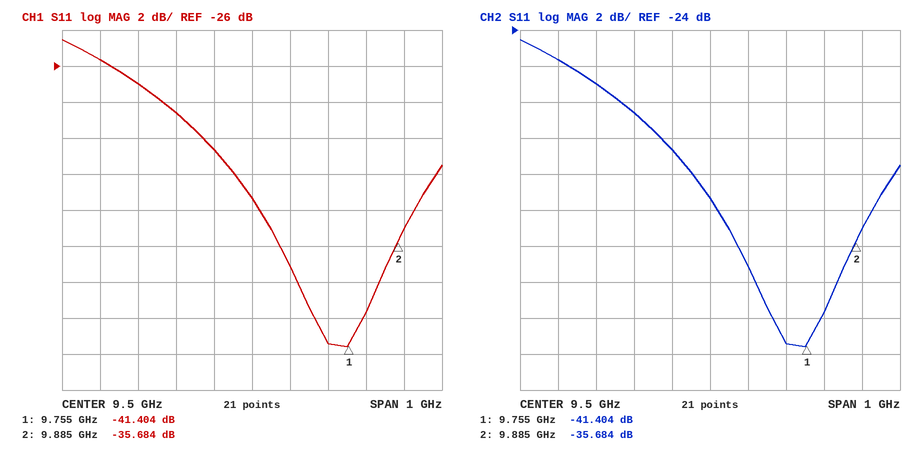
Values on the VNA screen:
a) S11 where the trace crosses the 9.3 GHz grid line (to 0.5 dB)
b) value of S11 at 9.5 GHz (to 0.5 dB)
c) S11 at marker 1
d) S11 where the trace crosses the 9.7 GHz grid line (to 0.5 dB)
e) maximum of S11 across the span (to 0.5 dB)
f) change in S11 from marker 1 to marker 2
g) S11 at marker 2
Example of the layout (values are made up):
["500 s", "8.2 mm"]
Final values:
["-28.5 dB", "-33.5 dB", "-41.404 dB", "-41.5 dB", "-24.5 dB", "5.720 dB", "-35.684 dB"]
